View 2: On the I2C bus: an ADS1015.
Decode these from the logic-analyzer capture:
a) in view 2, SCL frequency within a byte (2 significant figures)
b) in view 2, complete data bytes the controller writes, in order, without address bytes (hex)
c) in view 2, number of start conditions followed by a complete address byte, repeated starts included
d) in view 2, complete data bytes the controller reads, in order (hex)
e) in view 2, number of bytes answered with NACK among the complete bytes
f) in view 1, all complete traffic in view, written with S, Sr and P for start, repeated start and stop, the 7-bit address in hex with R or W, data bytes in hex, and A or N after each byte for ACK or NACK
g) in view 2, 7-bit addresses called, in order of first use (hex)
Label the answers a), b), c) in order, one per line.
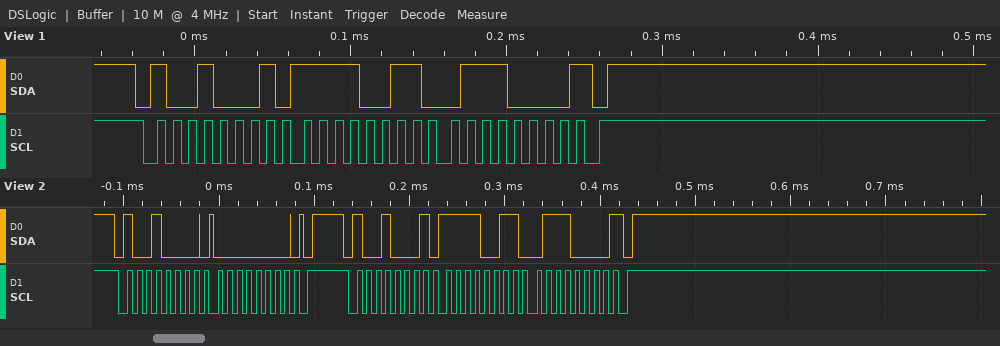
a) 100 kHz
b) 00
c) 2
d) F3 70
e) 1
f) S 48R A F3 A 70 N P
g) 0x48
